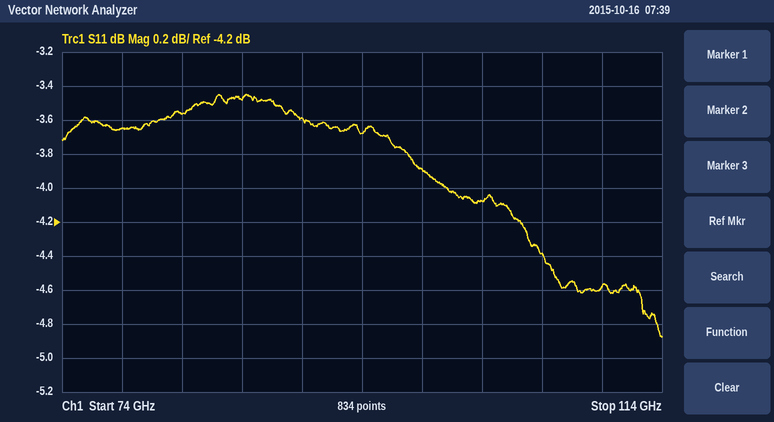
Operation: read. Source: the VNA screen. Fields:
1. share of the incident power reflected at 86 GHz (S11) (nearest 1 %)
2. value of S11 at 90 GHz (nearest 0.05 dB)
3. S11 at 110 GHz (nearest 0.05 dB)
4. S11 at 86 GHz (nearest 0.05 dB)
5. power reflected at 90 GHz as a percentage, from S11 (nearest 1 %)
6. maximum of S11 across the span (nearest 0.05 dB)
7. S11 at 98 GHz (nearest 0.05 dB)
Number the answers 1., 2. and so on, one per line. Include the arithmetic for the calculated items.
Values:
1. 10^(-3.5/10) ≈ 45 %
2. -3.60 dB
3. -4.60 dB
4. -3.50 dB
5. 10^(-3.6/10) ≈ 44 %
6. -3.45 dB
7. -3.90 dB
